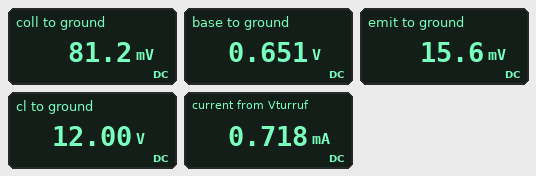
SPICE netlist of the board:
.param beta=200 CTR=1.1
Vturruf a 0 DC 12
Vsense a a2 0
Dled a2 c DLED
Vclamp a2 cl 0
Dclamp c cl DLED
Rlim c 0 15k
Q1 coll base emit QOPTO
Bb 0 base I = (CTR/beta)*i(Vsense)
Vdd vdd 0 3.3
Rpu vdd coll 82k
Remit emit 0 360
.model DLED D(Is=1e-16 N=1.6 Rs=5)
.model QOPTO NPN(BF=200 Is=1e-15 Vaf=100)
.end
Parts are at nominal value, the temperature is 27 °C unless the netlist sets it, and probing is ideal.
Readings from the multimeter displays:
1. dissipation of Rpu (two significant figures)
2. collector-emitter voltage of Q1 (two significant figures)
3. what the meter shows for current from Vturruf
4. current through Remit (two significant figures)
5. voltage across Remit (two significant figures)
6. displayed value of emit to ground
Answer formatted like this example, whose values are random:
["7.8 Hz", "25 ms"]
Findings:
["130 µW", "66 mV", "0.718 mA", "43 µA", "16 mV", "15.6 mV"]
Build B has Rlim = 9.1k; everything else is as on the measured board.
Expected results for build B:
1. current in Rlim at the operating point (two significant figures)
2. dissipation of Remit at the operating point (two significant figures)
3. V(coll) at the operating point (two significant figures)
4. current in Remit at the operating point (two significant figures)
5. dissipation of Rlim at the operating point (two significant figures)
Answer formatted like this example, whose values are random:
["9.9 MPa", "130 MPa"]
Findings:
["1.2 mA", "760 nW", "71 mV", "46 µA", "13 mW"]
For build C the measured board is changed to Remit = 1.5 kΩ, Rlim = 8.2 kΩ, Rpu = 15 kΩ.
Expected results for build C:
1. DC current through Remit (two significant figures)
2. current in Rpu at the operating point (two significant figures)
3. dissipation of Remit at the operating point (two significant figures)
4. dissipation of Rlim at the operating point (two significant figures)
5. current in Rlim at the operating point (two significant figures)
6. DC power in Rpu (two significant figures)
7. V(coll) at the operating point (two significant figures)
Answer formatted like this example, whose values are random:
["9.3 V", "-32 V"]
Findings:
["200 µA", "190 µA", "61 µW", "14 mW", "1.3 mA", "560 µW", "390 mV"]
